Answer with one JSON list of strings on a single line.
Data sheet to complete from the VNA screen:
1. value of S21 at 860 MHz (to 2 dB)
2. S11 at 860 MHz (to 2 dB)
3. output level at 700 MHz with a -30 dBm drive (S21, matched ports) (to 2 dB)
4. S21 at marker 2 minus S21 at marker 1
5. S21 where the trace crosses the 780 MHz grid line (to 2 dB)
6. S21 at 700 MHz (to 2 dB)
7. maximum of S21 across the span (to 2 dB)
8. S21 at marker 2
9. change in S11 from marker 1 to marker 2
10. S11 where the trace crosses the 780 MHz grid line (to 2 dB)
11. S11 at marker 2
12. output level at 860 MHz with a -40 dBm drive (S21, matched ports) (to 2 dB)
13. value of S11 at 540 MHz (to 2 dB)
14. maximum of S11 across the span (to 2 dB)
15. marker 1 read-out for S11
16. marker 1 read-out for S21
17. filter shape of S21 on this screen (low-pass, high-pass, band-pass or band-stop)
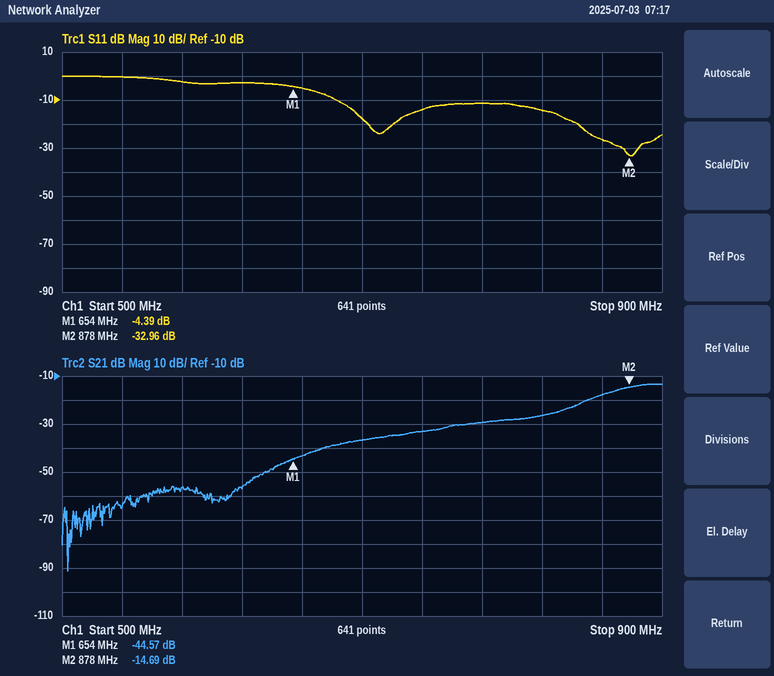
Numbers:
["-18 dB", "-26 dB", "-66 dBm", "29.88 dB", "-30 dB", "-36 dB", "-14 dB", "-14.69 dB", "-28.57 dB", "-12 dB", "-32.96 dB", "-58 dBm", "0 dB", "0 dB", "-4.39 dB", "-44.57 dB", "high-pass"]
